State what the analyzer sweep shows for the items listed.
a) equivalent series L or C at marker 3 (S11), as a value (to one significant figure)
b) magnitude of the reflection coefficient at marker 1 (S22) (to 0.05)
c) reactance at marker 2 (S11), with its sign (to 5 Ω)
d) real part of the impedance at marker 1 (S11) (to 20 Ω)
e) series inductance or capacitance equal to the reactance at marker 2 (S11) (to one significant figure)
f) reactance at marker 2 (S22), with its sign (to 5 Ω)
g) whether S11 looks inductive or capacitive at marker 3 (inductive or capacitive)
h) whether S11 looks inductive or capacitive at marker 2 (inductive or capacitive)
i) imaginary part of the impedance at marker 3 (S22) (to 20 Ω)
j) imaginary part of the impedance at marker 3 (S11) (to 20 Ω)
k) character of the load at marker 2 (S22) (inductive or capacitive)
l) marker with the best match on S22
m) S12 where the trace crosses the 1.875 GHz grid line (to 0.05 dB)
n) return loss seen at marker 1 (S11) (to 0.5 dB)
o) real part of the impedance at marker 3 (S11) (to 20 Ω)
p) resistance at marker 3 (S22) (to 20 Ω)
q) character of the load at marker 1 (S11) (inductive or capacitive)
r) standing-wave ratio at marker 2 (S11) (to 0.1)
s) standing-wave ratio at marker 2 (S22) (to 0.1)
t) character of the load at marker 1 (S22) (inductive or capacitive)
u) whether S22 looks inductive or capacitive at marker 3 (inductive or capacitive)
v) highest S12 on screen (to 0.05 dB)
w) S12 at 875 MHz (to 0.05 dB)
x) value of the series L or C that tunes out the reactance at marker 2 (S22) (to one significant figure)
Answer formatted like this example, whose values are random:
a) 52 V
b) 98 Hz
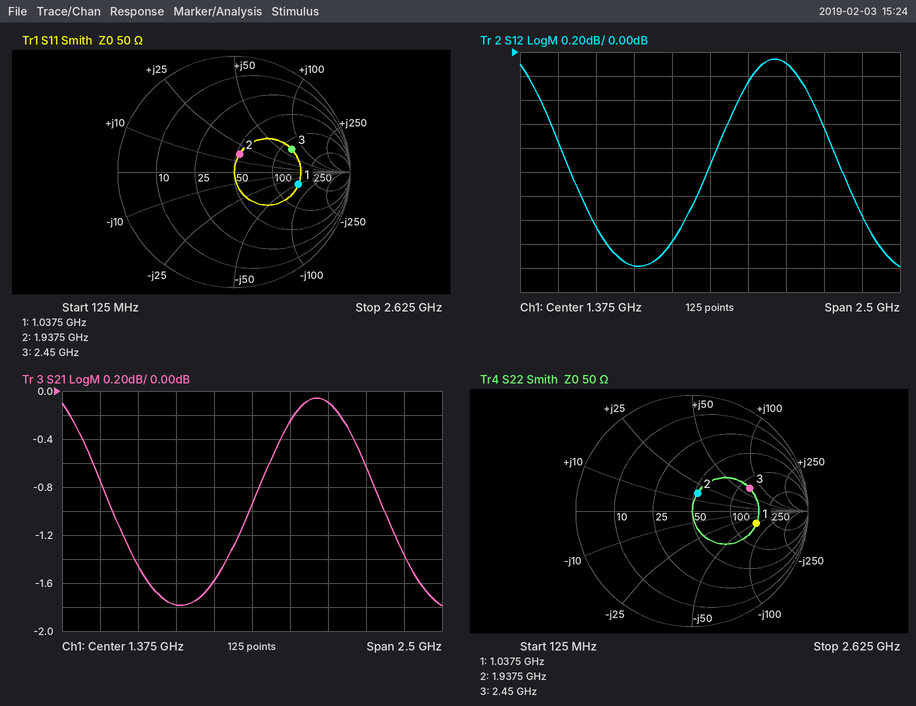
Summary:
a) 4 nH
b) 0.55
c) +15 Ω
d) 160 Ω
e) 1 nH
f) +15 Ω
g) inductive
h) inductive
i) +60 Ω
j) +60 Ω
k) inductive
l) marker 2
m) -0.10 dB
n) 5.0 dB
o) 120 Ω
p) 120 Ω
q) capacitive
r) 1.4
s) 1.4
t) capacitive
u) inductive
v) -0.05 dB
w) -1.80 dB
x) 5 pF
